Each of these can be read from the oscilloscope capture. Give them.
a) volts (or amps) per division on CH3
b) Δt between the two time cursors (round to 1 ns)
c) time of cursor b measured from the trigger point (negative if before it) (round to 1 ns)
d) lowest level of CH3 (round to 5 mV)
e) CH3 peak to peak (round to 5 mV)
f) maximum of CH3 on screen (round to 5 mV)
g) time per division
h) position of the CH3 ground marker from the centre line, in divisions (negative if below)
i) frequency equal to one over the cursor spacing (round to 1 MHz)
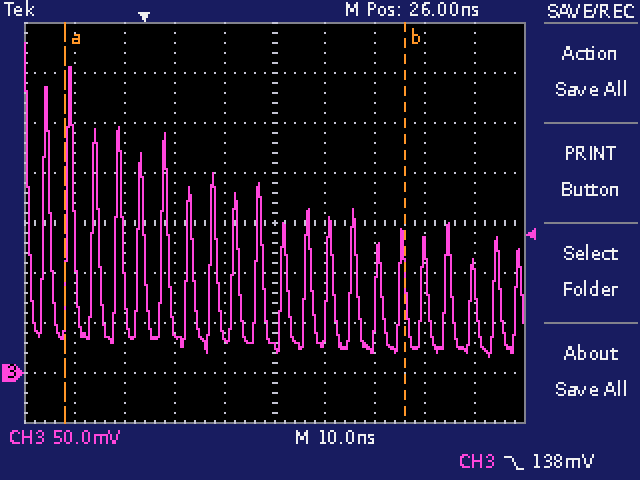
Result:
50 mV
68 ns
+52 ns
15 mV
315 mV
330 mV
10 ns
-3.0 div
15 MHz
